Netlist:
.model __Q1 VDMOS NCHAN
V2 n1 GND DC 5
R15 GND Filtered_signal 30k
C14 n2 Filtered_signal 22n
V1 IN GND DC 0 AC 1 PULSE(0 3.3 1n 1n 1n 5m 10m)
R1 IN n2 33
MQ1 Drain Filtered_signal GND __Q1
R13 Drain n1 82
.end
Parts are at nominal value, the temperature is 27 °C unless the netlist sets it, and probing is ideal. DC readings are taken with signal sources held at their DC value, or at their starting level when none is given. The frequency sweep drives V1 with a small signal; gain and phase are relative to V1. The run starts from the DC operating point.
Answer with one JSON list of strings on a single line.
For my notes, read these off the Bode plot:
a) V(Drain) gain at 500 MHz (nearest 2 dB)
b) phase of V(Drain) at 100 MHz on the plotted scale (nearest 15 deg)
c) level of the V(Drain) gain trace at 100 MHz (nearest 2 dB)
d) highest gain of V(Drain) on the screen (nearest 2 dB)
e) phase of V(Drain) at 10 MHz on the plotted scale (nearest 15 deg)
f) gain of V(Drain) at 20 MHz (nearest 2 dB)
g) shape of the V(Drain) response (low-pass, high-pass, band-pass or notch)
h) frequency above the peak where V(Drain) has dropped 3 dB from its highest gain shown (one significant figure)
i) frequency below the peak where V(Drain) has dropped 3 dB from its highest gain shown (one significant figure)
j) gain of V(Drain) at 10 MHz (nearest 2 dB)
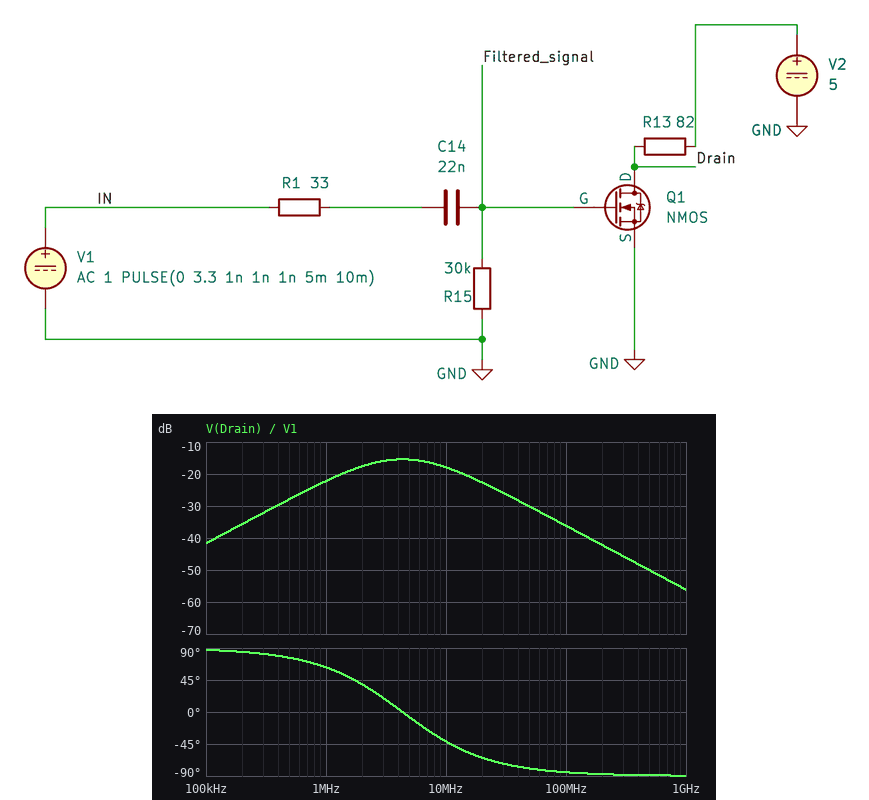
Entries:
["-50 dB", "-90 deg", "-36 dB", "-16 dB", "-45 deg", "-22 dB", "band-pass", "10 MHz", "2 MHz", "-18 dB"]
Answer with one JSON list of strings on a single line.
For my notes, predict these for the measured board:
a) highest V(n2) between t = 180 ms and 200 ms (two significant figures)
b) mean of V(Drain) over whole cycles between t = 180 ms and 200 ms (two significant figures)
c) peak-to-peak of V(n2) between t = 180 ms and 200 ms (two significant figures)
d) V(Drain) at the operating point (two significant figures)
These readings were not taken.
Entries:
["3.3 V", "5.0 V", "3.3 V", "5.0 V"]
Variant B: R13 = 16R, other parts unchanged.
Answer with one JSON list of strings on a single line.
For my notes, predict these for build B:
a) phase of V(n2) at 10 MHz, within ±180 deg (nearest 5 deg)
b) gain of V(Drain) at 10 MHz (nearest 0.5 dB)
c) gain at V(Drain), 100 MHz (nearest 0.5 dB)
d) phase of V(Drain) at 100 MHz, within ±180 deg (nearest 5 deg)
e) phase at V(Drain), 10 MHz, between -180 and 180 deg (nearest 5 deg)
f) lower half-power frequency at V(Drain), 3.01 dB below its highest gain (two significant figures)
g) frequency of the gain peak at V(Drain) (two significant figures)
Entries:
["-70 deg", "-26.5 dB", "-36.5 dB", "-70 deg", "0 deg", "2.7 MHz", "9.8 MHz"]
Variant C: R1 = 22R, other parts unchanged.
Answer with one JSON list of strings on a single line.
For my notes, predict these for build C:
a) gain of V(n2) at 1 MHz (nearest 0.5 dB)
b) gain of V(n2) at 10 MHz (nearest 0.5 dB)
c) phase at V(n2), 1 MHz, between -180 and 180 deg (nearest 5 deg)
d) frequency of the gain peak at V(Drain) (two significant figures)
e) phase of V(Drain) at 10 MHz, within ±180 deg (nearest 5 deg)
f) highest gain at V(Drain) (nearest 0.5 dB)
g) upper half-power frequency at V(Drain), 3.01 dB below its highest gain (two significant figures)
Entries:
["0 dB", "-7.0 dB", "-10 deg", "5.3 MHz", "-35 deg", "-13.5 dB", "13 MHz"]
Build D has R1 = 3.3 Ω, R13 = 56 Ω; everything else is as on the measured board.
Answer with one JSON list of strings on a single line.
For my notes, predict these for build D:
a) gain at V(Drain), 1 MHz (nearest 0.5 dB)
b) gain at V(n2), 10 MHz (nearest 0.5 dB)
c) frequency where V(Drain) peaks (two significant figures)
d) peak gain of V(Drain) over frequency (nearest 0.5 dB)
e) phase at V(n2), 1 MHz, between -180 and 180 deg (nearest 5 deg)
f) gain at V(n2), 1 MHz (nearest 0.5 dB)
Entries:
["-25.0 dB", "-0.5 dB", "17 MHz", "-9.0 dB", "0 deg", "0 dB"]
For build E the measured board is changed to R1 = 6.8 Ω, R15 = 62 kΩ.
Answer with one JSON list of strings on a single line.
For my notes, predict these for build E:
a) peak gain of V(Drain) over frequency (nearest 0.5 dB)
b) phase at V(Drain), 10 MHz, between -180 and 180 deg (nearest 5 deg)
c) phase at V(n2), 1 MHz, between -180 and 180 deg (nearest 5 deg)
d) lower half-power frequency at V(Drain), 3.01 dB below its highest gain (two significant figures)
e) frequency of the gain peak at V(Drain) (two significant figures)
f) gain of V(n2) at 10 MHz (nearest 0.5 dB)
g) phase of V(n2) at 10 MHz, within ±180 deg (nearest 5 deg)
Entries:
["-9.5 dB", "0 deg", "-5 deg", "3.5 MHz", "9.6 MHz", "-1.5 dB", "-30 deg"]
